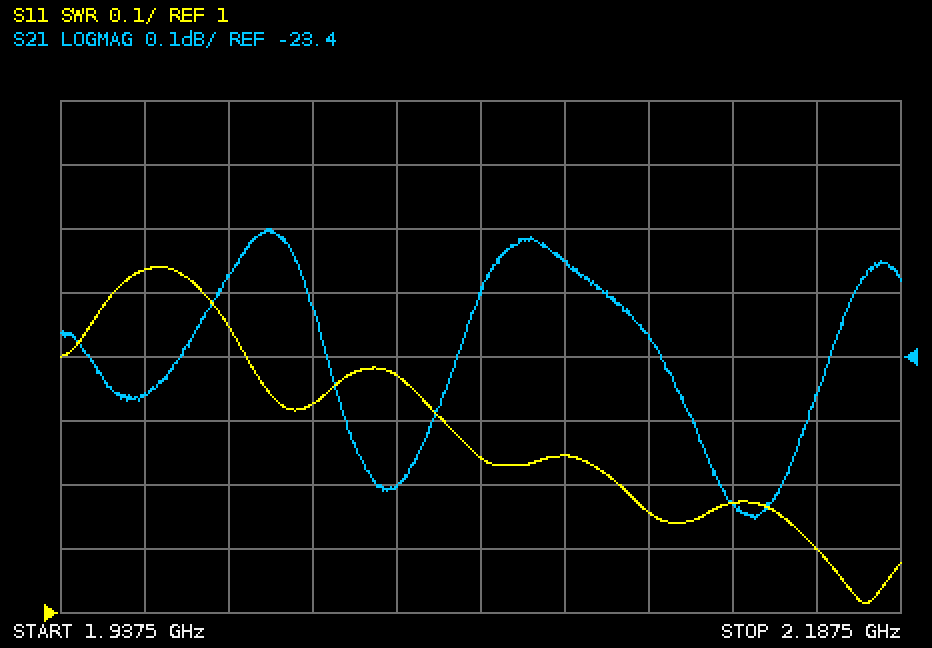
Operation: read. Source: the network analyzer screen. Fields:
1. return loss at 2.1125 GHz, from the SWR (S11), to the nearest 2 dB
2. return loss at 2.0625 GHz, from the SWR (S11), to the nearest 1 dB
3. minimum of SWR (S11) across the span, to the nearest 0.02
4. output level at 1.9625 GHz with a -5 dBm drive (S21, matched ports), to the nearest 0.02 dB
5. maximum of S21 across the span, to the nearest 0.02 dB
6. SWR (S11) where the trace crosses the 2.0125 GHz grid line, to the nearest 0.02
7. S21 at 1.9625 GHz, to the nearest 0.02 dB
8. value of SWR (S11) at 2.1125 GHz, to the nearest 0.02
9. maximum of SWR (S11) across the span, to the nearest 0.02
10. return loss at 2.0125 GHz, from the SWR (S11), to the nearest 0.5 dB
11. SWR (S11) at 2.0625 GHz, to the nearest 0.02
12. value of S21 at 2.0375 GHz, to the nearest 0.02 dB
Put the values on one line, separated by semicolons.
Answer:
22 dB; 19 dB; 1.02; -28.46 dBm; -23.20 dB; 1.32; -23.46 dB; 1.16; 1.54; 17.0 dB; 1.24; -23.60 dB
